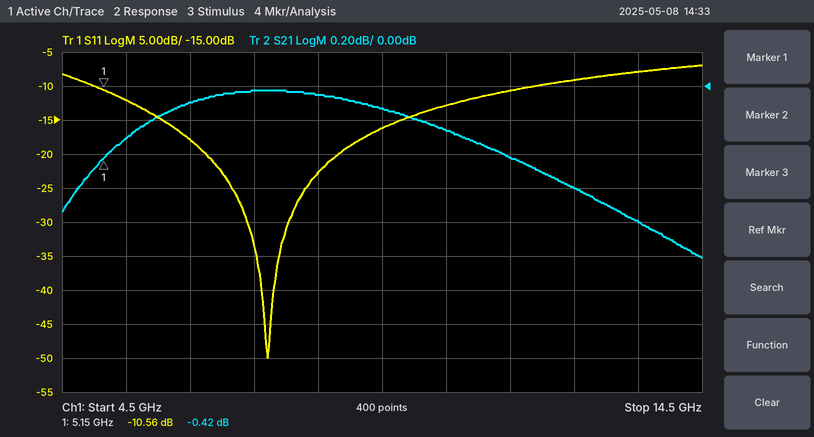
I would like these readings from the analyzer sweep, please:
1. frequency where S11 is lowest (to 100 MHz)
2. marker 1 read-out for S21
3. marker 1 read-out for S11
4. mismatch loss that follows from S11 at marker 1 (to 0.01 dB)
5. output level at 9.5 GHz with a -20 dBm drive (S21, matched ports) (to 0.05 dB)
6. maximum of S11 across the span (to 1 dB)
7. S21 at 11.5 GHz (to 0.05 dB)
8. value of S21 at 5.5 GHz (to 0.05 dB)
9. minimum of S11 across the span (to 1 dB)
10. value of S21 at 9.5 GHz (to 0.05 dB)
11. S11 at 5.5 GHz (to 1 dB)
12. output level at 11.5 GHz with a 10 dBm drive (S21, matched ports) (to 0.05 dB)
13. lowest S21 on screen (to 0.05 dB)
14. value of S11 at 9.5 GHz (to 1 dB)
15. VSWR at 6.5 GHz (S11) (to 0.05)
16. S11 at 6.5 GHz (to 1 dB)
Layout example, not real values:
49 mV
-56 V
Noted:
7.7 GHz
-0.42 dB
-10.56 dB
0.40 dB
-20.15 dBm
-7 dB
-0.40 dB
-0.30 dB
-50 dB
-0.15 dB
-12 dB
9.60 dBm
-1.00 dB
-16 dB
1.30
-18 dB
